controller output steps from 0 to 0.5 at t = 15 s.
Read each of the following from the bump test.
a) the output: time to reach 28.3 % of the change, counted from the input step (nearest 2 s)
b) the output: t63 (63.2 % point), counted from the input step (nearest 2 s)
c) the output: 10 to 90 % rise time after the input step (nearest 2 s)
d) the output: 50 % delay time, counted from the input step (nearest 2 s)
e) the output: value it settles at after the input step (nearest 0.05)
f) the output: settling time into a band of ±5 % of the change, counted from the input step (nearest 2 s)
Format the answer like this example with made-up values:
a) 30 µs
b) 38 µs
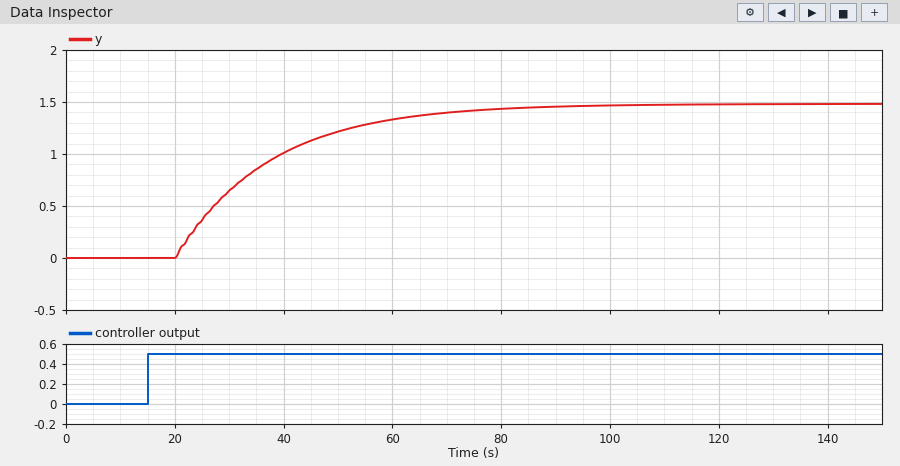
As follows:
a) 10 s
b) 22 s
c) 38 s
d) 18 s
e) 1.50
f) 58 s
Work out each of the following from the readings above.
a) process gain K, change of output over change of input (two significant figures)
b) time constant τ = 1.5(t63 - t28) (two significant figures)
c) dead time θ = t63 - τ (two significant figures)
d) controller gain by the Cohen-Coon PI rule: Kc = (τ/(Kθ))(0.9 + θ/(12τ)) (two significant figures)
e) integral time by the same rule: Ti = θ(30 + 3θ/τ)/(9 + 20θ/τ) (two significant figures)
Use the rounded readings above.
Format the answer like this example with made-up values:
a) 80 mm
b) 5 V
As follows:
a) 3.0
b) 18 s
c) 4.0 s
d) 1.4
e) 9.1 s
